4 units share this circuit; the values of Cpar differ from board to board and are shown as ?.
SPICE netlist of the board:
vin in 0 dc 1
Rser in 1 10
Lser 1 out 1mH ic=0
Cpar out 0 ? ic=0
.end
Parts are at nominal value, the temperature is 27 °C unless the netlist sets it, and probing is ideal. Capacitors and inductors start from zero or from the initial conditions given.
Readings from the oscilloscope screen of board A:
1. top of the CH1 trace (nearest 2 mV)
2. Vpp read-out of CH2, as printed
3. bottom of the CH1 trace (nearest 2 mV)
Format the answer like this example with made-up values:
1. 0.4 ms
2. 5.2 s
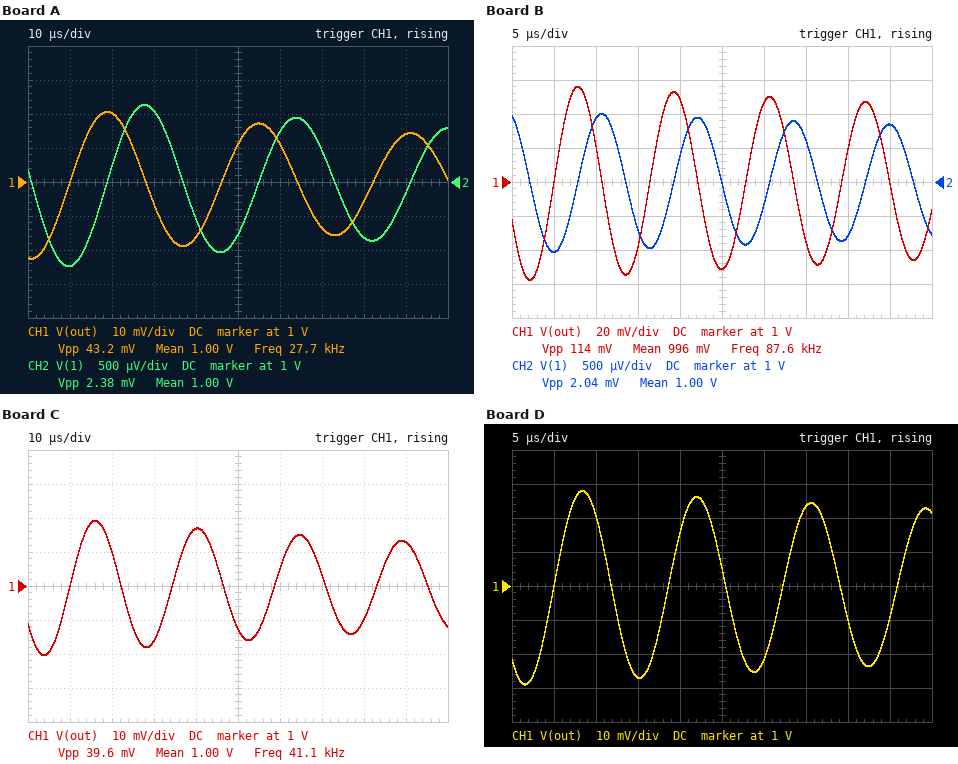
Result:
1. 1.020 V
2. 2.38 mV
3. 978 mV
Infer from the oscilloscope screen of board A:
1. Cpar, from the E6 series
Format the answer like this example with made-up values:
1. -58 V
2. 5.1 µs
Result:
1. 33 nF
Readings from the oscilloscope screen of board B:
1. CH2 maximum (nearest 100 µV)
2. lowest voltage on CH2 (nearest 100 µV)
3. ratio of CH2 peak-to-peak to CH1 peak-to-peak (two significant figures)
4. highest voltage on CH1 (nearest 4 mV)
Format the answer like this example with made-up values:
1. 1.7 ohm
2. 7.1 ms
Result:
1. 1.0010 V
2. 999.0 mV
3. 0.018
4. 1.056 V
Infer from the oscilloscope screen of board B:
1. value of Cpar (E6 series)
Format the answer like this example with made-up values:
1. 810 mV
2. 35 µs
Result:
1. 3.3 nF
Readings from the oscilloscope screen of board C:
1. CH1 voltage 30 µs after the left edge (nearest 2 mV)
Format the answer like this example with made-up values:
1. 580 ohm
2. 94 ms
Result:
1. 984 mV
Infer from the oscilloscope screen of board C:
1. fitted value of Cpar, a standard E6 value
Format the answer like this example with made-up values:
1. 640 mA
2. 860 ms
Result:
1. 15 nF
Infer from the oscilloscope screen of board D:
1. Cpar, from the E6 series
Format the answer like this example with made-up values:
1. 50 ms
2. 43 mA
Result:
1. 4.7 nF
